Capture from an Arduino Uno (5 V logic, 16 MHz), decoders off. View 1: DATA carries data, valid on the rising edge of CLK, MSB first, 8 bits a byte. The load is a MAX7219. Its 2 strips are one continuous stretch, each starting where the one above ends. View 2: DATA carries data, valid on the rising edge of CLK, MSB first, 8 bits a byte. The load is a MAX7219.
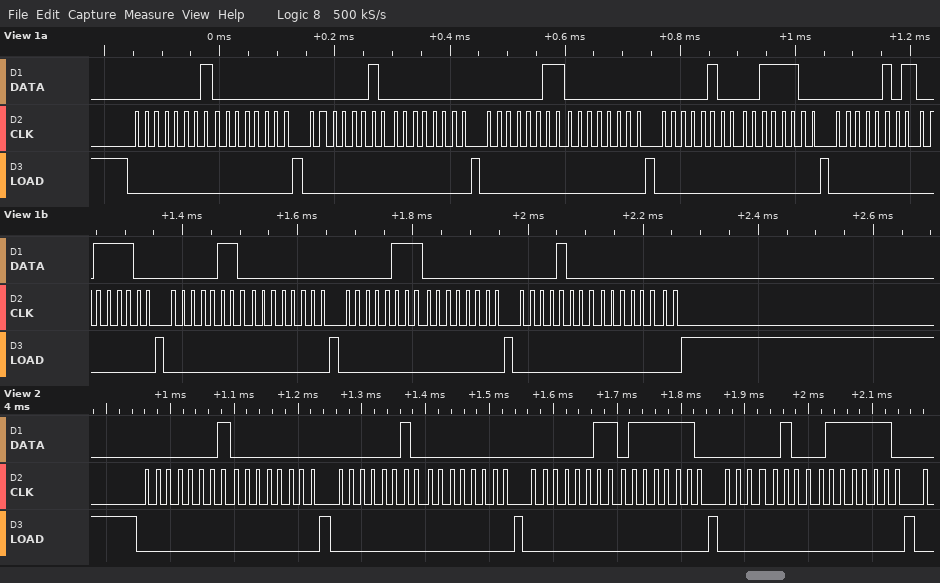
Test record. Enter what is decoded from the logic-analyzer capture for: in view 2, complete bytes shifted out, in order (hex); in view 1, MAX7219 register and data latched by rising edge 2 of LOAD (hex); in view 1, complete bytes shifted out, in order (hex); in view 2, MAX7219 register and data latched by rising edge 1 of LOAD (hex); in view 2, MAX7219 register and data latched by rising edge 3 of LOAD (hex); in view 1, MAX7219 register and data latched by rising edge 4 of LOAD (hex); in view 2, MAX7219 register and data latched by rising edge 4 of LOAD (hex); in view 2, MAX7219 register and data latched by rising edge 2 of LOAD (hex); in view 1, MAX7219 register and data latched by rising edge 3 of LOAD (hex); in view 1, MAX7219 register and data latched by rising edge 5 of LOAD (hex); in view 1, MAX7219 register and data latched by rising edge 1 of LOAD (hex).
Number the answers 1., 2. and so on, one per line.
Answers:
1. 0x01 0x00 0x02 0x00 0x03 0x7E 0x04 0x7E
2. register 0x2, data 0x00
3. 0x01 0x00 0x02 0x00 0x03 0x00 0x04 0x3C 0x05 0x3C 0x06 0x00 0x07 0x00 0x08 0x00
4. register 0x1, data 0x00
5. register 0x3, data 0x7E
6. register 0x4, data 0x3C
7. register 0x4, data 0x7E
8. register 0x2, data 0x00
9. register 0x3, data 0x00
10. register 0x5, data 0x3C
11. register 0x1, data 0x00
